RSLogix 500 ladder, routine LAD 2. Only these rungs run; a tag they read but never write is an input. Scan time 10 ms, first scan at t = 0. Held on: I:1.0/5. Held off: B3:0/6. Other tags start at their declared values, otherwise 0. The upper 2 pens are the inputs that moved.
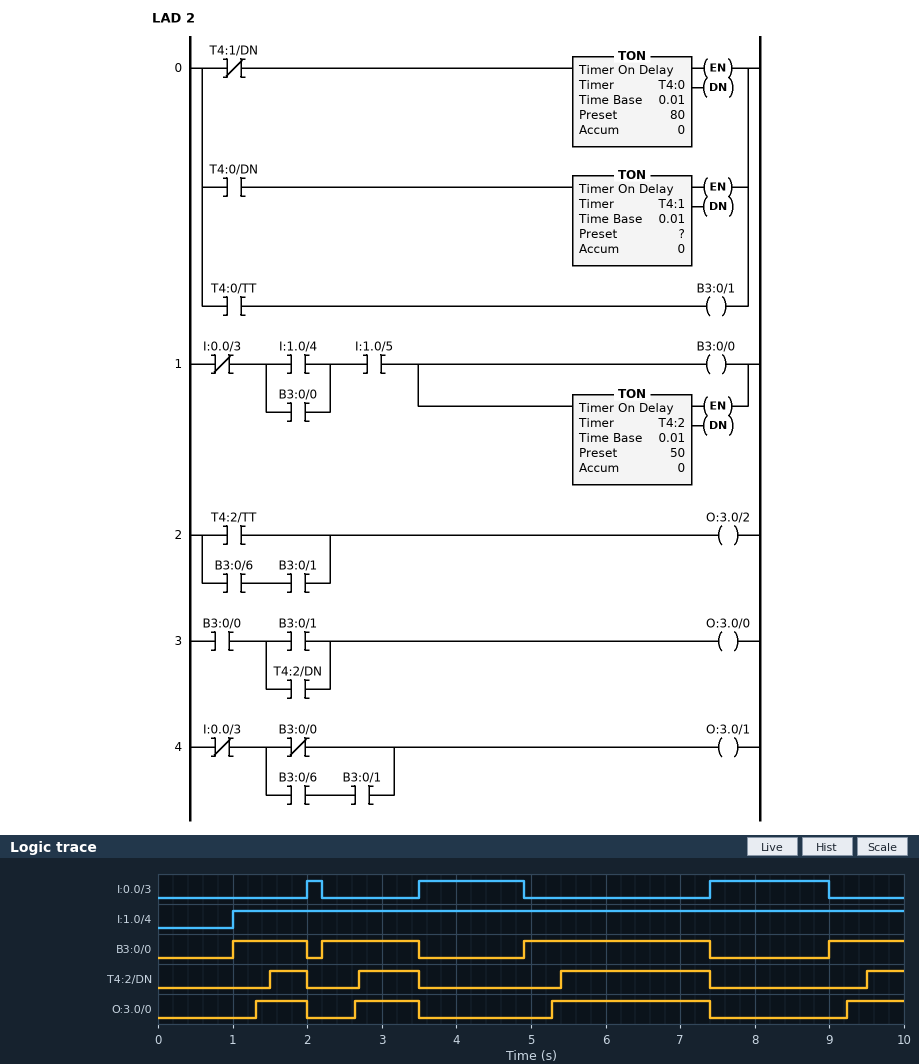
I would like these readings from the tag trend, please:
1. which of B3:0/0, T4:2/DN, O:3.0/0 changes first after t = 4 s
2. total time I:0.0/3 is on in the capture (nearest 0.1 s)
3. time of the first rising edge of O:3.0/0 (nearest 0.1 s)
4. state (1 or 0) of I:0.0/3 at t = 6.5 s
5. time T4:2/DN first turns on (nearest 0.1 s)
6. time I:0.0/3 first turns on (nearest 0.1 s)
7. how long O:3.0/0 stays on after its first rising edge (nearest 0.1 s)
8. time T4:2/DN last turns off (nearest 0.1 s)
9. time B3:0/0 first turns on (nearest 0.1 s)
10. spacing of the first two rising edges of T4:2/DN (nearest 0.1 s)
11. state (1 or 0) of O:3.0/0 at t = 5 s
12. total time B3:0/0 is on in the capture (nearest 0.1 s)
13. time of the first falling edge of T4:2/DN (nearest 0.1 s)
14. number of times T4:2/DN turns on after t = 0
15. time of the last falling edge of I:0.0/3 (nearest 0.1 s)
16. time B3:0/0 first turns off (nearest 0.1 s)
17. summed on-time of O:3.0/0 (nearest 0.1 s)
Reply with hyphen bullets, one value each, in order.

- B3:0/0
- 3.2 s
- 1.3 s
- 0
- 1.5 s
- 2.0 s
- 0.7 s
- 7.4 s
- 1.0 s
- 1.2 s
- 0
- 5.8 s
- 2.0 s
- 4
- 9.0 s
- 2.0 s
- 4.4 s
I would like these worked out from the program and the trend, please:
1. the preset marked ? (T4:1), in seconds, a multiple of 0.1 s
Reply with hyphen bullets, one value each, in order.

- 0.5 s
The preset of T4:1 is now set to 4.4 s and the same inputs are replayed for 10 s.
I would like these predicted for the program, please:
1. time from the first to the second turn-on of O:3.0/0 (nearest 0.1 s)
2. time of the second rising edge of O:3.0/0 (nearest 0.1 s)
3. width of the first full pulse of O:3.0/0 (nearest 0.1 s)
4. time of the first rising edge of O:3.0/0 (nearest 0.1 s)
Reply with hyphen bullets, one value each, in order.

- 1.2 s
- 2.7 s
- 0.5 s
- 1.5 s
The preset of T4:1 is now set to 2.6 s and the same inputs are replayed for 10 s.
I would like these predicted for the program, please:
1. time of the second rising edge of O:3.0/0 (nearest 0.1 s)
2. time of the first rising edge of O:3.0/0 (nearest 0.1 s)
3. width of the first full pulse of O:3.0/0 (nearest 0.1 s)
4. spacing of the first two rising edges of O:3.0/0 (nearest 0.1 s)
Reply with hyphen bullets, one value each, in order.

- 2.7 s
- 1.5 s
- 0.5 s
- 1.2 s
